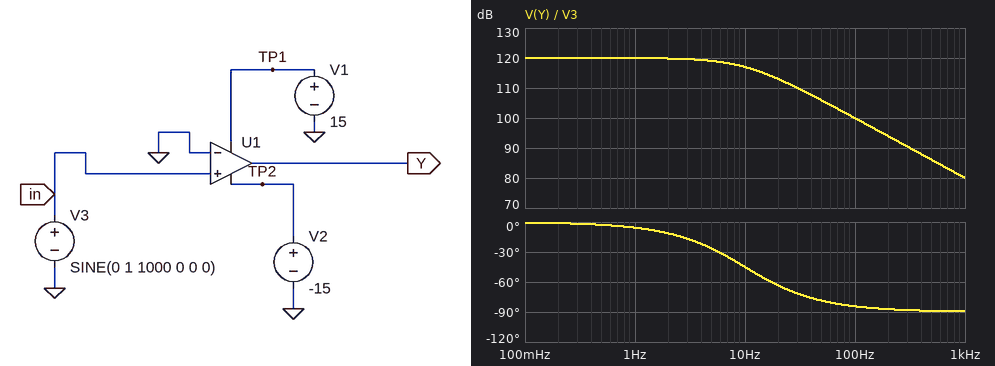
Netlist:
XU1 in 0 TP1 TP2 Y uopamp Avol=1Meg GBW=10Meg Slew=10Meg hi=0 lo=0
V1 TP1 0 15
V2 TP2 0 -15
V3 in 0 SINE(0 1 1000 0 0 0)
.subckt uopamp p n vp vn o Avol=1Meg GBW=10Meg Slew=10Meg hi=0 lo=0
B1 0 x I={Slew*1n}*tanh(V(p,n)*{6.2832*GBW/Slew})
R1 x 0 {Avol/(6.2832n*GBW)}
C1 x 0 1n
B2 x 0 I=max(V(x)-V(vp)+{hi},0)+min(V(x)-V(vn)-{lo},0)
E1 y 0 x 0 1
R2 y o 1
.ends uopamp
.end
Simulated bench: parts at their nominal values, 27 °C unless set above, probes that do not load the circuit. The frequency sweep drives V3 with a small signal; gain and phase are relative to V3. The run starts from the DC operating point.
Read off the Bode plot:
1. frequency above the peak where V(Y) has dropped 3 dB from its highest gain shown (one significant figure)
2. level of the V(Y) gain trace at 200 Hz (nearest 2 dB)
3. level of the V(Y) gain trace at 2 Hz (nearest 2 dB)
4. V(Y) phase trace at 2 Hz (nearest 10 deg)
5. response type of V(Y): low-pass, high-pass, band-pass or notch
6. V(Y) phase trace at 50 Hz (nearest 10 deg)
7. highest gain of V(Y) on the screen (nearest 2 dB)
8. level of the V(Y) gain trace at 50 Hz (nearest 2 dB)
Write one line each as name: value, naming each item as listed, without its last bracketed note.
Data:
frequency above the peak where V(Y) has dropped 3 dB from its highest gain shown: 10 Hz
level of the V(Y) gain trace at 200 Hz: 94 dB
level of the V(Y) gain trace at 2 Hz: 120 dB
V(Y) phase trace at 2 Hz: -10 deg
response type of V(Y): low-pass, high-pass, band-pass or notch: low-pass
V(Y) phase trace at 50 Hz: -80 deg
highest gain of V(Y) on the screen: 120 dB
level of the V(Y) gain trace at 50 Hz: 106 dB
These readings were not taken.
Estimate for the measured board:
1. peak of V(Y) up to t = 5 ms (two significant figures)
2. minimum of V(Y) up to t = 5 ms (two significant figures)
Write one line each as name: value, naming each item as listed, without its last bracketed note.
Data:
peak of V(Y) up to t = 5 ms: 15 V
minimum of V(Y) up to t = 5 ms: -15 V
